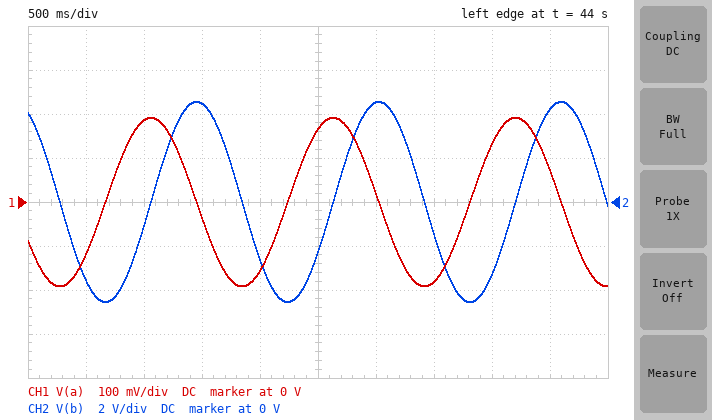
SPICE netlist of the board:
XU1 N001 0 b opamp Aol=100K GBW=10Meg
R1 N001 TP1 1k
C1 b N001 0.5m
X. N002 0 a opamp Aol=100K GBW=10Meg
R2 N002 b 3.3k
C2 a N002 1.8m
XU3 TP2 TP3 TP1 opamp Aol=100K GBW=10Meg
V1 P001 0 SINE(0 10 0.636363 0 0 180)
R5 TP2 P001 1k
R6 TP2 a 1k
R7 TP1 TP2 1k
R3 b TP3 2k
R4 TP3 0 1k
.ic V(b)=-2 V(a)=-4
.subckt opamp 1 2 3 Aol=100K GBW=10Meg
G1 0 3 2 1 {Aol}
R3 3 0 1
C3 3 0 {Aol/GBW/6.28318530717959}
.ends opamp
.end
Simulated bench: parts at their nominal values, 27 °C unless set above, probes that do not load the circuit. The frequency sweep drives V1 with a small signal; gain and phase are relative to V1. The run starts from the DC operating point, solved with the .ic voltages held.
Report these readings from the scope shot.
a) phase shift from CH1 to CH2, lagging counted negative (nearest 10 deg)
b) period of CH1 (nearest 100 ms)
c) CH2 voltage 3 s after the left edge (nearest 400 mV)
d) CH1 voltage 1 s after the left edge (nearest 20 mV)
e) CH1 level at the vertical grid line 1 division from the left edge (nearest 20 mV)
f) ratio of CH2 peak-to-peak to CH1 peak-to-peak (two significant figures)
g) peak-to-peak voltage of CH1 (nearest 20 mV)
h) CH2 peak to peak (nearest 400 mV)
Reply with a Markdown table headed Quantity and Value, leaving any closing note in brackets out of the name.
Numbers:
| Quantity | Value |
|---|---|
| phase shift from CH1 to CH2, lagging counted negative | -90 deg |
| period of CH1 | 1.6 s |
| CH2 voltage 3 s after the left edge | 4.4 V |
| CH1 voltage 1 s after the left edge | 180 mV |
| CH1 level at the vertical grid line 1 division from the left edge | -120 mV |
| ratio of CH2 peak-to-peak to CH1 peak-to-peak | 24 |
| peak-to-peak voltage of CH1 | 380 mV |
| CH2 peak to peak | 9.2 V |
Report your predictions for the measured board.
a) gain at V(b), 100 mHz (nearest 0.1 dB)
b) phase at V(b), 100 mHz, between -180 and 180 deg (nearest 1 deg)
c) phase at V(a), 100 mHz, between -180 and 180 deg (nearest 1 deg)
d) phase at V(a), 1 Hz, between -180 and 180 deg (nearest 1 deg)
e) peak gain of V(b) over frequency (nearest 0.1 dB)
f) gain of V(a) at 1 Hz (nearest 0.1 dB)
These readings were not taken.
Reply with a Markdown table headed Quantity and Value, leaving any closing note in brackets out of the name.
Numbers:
| Quantity | Value |
|---|---|
| gain at V(b), 100 mHz | 0 dB |
| phase at V(b), 100 mHz, between -180 and 180 deg | -3 deg |
| phase at V(a), 100 mHz, between -180 and 180 deg | 87 deg |
| phase at V(a), 1 Hz, between -180 and 180 deg | 18 deg |
| peak gain of V(b) over frequency | 0 dB |
| gain of V(a) at 1 Hz | -41.7 dB |
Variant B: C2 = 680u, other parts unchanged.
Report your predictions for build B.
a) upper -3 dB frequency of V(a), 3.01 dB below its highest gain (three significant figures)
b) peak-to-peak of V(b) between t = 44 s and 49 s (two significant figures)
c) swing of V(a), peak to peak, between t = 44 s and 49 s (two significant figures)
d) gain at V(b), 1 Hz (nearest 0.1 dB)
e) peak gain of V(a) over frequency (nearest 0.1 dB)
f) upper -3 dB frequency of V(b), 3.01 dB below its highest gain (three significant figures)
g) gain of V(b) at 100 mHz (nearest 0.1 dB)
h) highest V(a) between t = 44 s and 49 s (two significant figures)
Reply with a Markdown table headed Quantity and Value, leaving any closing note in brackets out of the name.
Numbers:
| Quantity | Value |
|---|---|
| upper -3 dB frequency of V(a), 3.01 dB below its highest gain | 89.2 mHz |
| peak-to-peak of V(b) between t = 44 s and 49 s | 9.4 V |
| swing of V(a), peak to peak, between t = 44 s and 49 s | 1.0 V |
| gain at V(b), 1 Hz | -10.2 dB |
| peak gain of V(a) over frequency | 0 dB |
| upper -3 dB frequency of V(b), 3.01 dB below its highest gain | 378 mHz |
| gain of V(b) at 100 mHz | -0.6 dB |
| highest V(a) between t = 44 s and 49 s | 520 mV |
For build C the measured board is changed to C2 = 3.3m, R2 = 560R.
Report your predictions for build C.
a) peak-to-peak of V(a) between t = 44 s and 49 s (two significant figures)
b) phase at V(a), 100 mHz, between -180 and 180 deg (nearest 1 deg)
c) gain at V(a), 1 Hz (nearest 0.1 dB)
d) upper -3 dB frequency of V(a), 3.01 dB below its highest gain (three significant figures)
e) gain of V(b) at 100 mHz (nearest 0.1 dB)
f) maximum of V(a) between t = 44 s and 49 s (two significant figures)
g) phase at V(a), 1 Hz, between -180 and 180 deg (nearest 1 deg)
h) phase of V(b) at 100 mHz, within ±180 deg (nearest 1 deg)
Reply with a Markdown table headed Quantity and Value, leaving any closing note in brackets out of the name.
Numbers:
| Quantity | Value |
|---|---|
| peak-to-peak of V(a) between t = 44 s and 49 s | 1.3 V |
| phase at V(a), 100 mHz, between -180 and 180 deg | 119 deg |
| gain at V(a), 1 Hz | -31.4 dB |
| upper -3 dB frequency of V(a), 3.01 dB below its highest gain | 113 mHz |
| gain of V(b) at 100 mHz | -1.1 dB |
| maximum of V(a) between t = 44 s and 49 s | 640 mV |
| phase at V(a), 1 Hz, between -180 and 180 deg | 18 deg |
| phase of V(b) at 100 mHz, within ±180 deg | 29 deg |
